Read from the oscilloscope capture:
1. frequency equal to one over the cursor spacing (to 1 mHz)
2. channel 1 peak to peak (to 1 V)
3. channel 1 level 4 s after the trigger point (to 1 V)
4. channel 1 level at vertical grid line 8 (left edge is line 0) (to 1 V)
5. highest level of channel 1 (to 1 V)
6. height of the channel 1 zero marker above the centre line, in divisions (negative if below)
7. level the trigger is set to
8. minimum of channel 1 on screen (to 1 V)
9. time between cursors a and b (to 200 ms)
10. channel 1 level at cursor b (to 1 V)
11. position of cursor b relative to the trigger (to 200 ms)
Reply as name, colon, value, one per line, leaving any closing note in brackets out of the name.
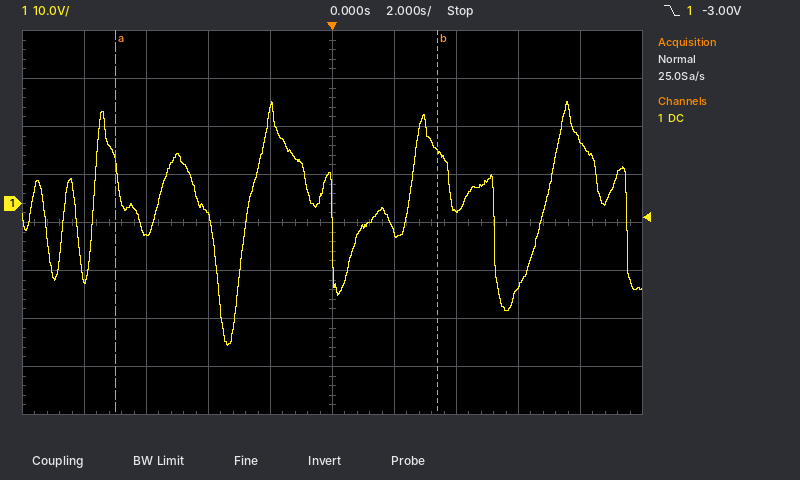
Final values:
frequency equal to one over the cursor spacing: 96 mHz
channel 1 peak to peak: 51 V
channel 1 level 4 s after the trigger point: -2 V
channel 1 level at vertical grid line 8 (left edge is line 0): -17 V
highest level of channel 1: 21 V
height of the channel 1 zero marker above the centre line, in divisions: +0.4 div
level the trigger is set to: -3.00 V
minimum of channel 1 on screen: -30 V
time between cursors a and b: 10.4 s
channel 1 level at cursor b: 11 V
position of cursor b relative to the trigger: +3.4 s
